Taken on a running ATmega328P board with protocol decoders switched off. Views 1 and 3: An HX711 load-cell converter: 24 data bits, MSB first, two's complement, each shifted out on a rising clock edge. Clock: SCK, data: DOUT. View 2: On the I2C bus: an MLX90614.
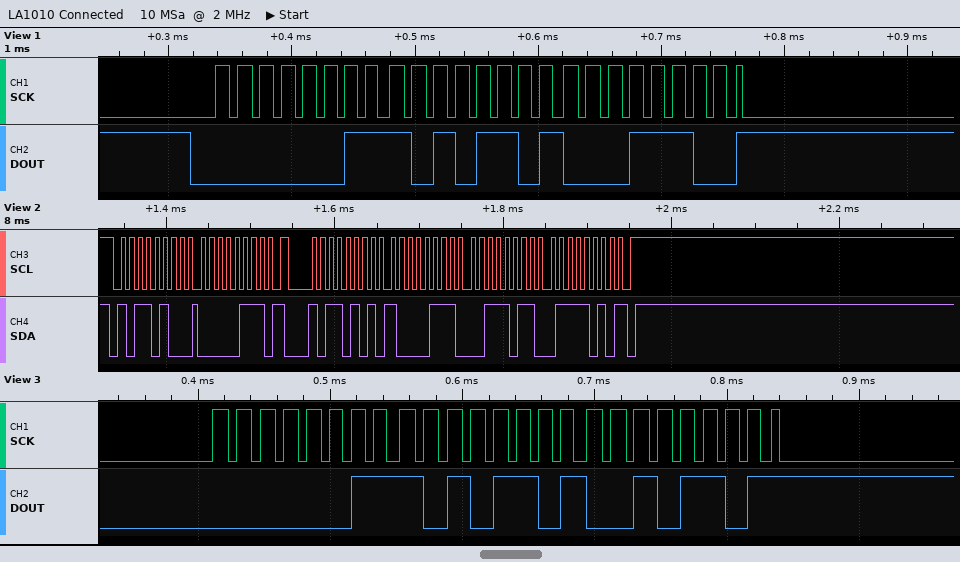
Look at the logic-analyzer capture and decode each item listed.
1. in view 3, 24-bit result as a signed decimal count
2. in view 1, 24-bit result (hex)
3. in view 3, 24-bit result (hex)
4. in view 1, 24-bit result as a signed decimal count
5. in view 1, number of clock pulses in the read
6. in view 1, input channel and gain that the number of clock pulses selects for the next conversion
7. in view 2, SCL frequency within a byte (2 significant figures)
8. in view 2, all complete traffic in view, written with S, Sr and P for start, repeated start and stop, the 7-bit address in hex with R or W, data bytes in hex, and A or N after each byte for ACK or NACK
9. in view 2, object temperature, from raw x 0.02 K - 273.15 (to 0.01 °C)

240941
0x03AD1C
0x03AD2D
240924
25
channel A, gain 128
100 kHz
S 5AW A 07 A Sr 5AR A 87 A 3B A 7A N P
31.63 °C
